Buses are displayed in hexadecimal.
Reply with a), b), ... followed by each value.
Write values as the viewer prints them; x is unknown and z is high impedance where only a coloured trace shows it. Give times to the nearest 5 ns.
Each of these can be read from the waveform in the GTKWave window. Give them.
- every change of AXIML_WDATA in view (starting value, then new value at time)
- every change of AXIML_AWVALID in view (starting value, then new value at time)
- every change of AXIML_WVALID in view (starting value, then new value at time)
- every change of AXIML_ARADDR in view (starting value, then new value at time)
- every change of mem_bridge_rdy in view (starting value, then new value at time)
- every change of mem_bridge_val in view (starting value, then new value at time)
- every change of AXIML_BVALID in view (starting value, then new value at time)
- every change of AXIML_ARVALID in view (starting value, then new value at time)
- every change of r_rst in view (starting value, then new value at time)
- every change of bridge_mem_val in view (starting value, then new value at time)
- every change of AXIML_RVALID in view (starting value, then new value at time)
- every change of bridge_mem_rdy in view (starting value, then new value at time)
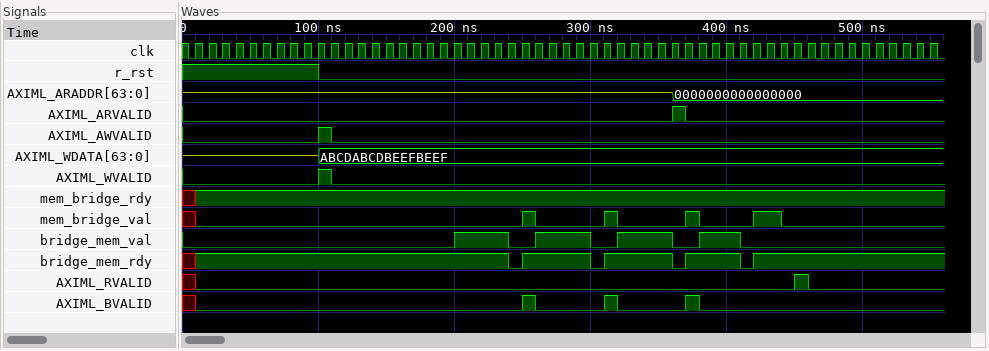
a) z, ABCDABCDBEEFBEEF at 100 ns
b) 0, 1 at 100 ns, 0 at 110 ns
c) 0, 1 at 100 ns, 0 at 110 ns
d) z, 0000000000000000 at 360 ns
e) x, 1 at 10 ns
f) x, 0 at 10 ns, 1 at 250 ns, 0 at 260 ns, 1 at 310 ns, 0 at 320 ns, 1 at 370 ns, 0 at 380 ns, 1 at 420 ns, 0 at 440 ns
g) x, 0 at 10 ns, 1 at 250 ns, 0 at 260 ns, 1 at 310 ns, 0 at 320 ns, 1 at 370 ns, 0 at 380 ns
h) 0, 1 at 360 ns, 0 at 370 ns
i) 1, 0 at 100 ns
j) 0, 1 at 200 ns, 0 at 240 ns, 1 at 260 ns, 0 at 300 ns, 1 at 320 ns, 0 at 360 ns, 1 at 380 ns, 0 at 410 ns
k) x, 0 at 10 ns, 1 at 450 ns, 0 at 460 ns
l) x, 1 at 10 ns, 0 at 240 ns, 1 at 250 ns, 0 at 300 ns, 1 at 310 ns, 0 at 360 ns, 1 at 370 ns, 0 at 410 ns, 1 at 420 ns
